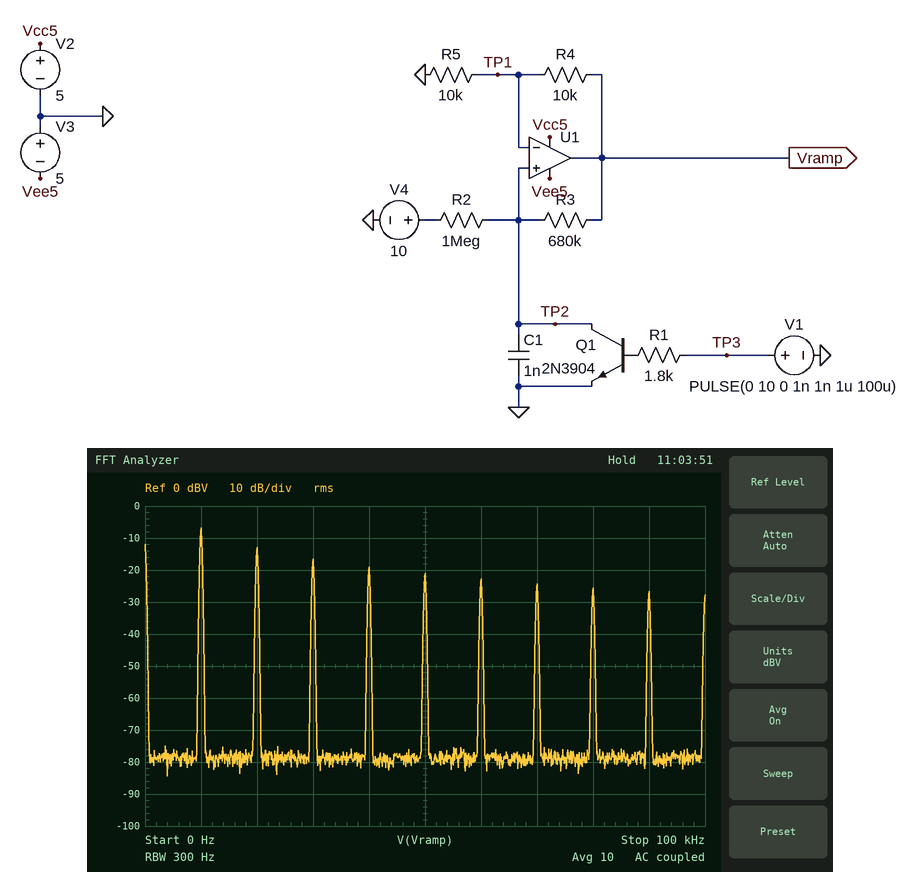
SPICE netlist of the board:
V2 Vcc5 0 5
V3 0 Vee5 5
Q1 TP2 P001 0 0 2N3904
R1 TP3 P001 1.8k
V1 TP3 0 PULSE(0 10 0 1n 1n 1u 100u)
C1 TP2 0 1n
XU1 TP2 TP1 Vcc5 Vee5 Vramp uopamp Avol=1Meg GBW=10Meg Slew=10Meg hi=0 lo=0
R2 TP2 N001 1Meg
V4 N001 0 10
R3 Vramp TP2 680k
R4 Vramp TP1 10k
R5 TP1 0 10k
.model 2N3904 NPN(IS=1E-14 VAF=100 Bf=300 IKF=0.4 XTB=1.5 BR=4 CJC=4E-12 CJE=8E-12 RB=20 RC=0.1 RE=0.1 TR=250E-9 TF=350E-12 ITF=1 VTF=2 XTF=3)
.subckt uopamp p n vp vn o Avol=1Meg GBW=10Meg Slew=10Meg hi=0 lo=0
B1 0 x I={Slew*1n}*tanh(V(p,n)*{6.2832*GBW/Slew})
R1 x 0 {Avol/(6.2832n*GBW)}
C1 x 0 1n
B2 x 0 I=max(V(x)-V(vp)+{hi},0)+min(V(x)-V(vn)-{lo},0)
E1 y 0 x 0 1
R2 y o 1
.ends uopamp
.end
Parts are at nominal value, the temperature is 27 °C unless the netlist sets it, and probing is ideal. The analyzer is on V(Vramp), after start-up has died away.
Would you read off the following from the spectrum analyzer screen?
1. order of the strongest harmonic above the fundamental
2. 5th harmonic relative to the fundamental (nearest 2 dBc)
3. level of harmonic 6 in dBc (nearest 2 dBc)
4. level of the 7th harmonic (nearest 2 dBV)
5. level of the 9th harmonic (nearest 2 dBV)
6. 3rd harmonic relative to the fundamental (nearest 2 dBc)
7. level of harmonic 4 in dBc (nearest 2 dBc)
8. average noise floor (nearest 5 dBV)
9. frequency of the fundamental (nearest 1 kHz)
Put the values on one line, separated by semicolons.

2; -14 dBc; -16 dBc; -24 dBV; -26 dBV; -10 dBc; -12 dBc; -80 dBV; 10 kHz
